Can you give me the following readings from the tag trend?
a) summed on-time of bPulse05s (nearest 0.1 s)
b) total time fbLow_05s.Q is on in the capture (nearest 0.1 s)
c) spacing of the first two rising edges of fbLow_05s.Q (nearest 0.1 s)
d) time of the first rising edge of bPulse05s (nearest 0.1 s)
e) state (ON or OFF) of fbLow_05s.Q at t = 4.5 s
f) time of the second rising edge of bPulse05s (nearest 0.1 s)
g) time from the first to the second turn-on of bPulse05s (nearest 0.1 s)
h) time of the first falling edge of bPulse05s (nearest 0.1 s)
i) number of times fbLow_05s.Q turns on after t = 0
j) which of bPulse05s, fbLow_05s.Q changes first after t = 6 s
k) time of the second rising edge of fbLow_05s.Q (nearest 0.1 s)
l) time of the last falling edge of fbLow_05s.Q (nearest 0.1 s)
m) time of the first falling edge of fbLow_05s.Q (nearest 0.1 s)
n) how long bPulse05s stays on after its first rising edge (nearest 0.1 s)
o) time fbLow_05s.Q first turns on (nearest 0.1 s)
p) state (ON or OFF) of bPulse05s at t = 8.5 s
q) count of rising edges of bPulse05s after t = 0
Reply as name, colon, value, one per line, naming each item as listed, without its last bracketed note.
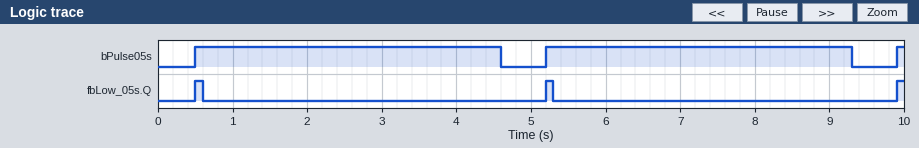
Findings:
summed on-time of bPulse05s: 8.3 s
total time fbLow_05s.Q is on in the capture: 0.3 s
spacing of the first two rising edges of fbLow_05s.Q: 4.7 s
time of the first rising edge of bPulse05s: 0.5 s
state (ON or OFF) of fbLow_05s.Q at t = 4.5 s: OFF
time of the second rising edge of bPulse05s: 5.2 s
time from the first to the second turn-on of bPulse05s: 4.7 s
time of the first falling edge of bPulse05s: 4.6 s
number of times fbLow_05s.Q turns on after t = 0: 3
which of bPulse05s, fbLow_05s.Q changes first after t = 6 s: bPulse05s
time of the second rising edge of fbLow_05s.Q: 5.2 s
time of the last falling edge of fbLow_05s.Q: 5.3 s
time of the first falling edge of fbLow_05s.Q: 0.6 s
how long bPulse05s stays on after its first rising edge: 4.1 s
time fbLow_05s.Q first turns on: 0.5 s
state (ON or OFF) of bPulse05s at t = 8.5 s: ON
count of rising edges of bPulse05s after t = 0: 3
